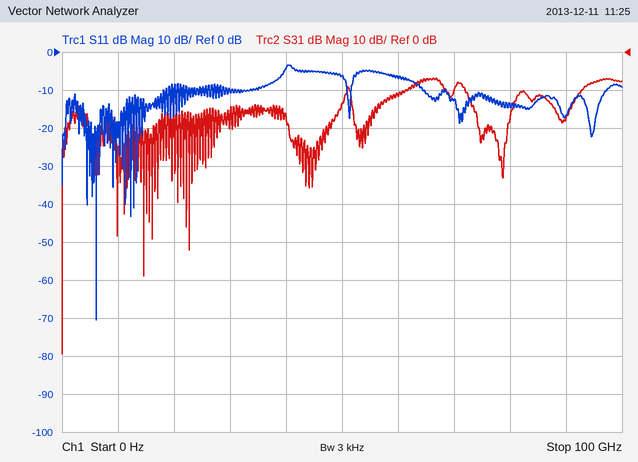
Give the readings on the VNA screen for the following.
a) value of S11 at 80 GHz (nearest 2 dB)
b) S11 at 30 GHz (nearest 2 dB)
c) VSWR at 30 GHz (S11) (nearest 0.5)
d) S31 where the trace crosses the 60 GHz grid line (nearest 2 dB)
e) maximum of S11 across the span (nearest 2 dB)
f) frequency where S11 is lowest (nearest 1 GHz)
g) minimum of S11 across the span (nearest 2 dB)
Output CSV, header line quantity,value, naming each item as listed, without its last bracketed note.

quantity,value
value of S11 at 80 GHz,-14 dB
S11 at 30 GHz,-10 dB
VSWR at 30 GHz (S11),2.0
S31 where the trace crosses the 60 GHz grid line,-12 dB
maximum of S11 across the span,-4 dB
frequency where S11 is lowest,6 GHz
minimum of S11 across the span,-70 dB
